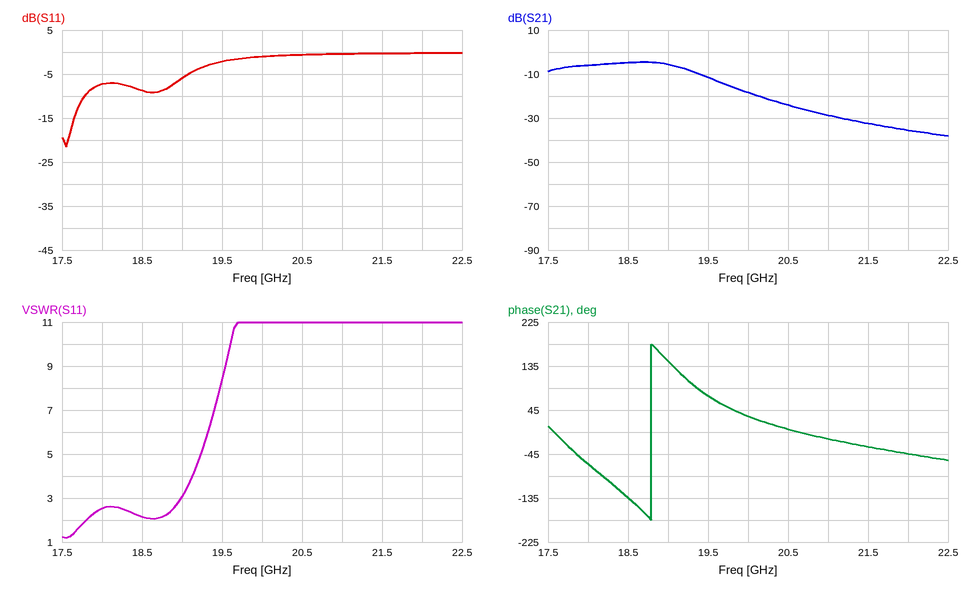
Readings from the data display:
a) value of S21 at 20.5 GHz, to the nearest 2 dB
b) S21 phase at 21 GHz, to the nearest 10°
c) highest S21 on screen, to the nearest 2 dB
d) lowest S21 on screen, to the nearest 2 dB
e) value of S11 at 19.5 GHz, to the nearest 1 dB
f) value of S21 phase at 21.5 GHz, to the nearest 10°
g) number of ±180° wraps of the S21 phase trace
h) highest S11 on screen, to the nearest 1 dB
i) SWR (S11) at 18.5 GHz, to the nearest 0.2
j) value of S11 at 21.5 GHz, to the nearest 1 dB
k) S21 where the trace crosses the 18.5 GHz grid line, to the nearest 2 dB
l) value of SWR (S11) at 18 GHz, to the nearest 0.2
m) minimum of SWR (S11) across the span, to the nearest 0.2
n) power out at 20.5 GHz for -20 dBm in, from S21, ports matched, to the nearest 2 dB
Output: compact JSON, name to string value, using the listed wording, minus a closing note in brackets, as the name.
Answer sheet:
{"value of S21 at 20.5 GHz, to the nearest 2 dB": "-24 dB", "S21 phase at 21 GHz, to the nearest 10°": "-10°", "highest S21 on screen, to the nearest 2 dB": "-4 dB", "lowest S21 on screen, to the nearest 2 dB": "-38 dB", "value of S11 at 19.5 GHz, to the nearest 1 dB": "-2 dB", "value of S21 phase at 21.5 GHz, to the nearest 10°": "-30°", "number of ±180° wraps of the S21 phase trace": "1", "highest S11 on screen, to the nearest 1 dB": "0 dB", "SWR (S11) at 18.5 GHz, to the nearest 0.2": "2.2", "value of S11 at 21.5 GHz, to the nearest 1 dB": "0 dB", "S21 where the trace crosses the 18.5 GHz grid line, to the nearest 2 dB": "-4 dB", "value of SWR (S11) at 18 GHz, to the nearest 0.2": "2.6", "minimum of SWR (S11) across the span, to the nearest 0.2": "1.2", "power out at 20.5 GHz for -20 dBm in, from S21, ports matched, to the nearest 2 dB": "-44 dBm"}
